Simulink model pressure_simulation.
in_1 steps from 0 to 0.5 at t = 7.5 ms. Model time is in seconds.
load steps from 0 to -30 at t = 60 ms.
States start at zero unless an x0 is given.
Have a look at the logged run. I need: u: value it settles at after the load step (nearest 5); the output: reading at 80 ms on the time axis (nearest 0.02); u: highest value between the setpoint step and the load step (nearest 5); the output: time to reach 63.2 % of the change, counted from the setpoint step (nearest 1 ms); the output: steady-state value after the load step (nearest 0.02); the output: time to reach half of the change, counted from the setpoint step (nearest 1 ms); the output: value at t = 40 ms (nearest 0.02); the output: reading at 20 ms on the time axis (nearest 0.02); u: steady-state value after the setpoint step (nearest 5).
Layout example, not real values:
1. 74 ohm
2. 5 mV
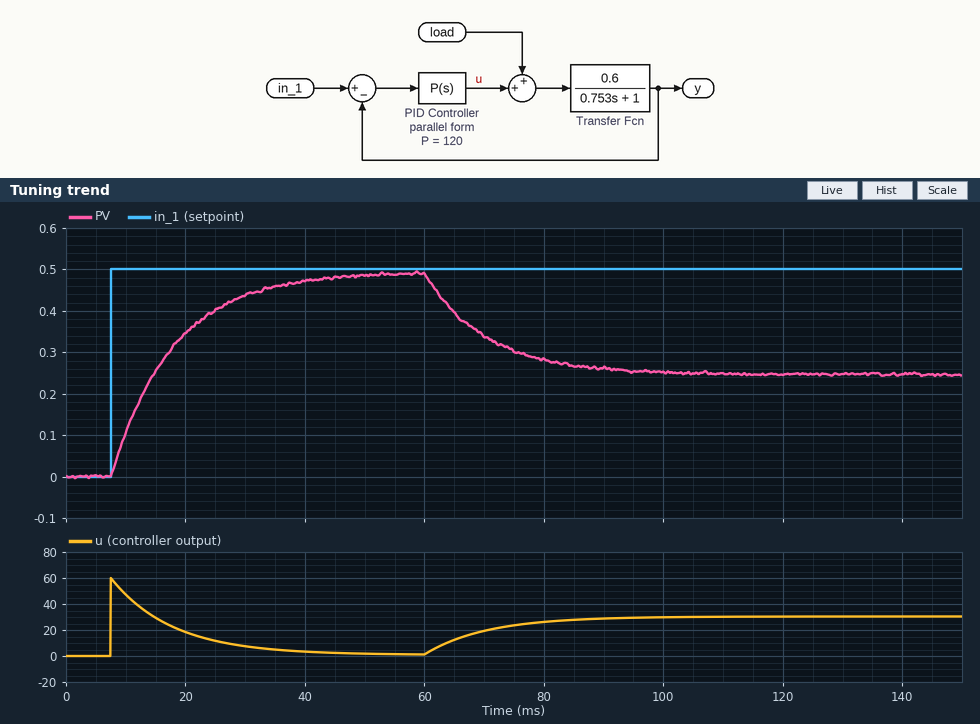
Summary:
1. 30
2. 0.28
3. 60
4. 10 ms
5. 0.24
6. 7 ms
7. 0.48
8. 0.34
9. 0
